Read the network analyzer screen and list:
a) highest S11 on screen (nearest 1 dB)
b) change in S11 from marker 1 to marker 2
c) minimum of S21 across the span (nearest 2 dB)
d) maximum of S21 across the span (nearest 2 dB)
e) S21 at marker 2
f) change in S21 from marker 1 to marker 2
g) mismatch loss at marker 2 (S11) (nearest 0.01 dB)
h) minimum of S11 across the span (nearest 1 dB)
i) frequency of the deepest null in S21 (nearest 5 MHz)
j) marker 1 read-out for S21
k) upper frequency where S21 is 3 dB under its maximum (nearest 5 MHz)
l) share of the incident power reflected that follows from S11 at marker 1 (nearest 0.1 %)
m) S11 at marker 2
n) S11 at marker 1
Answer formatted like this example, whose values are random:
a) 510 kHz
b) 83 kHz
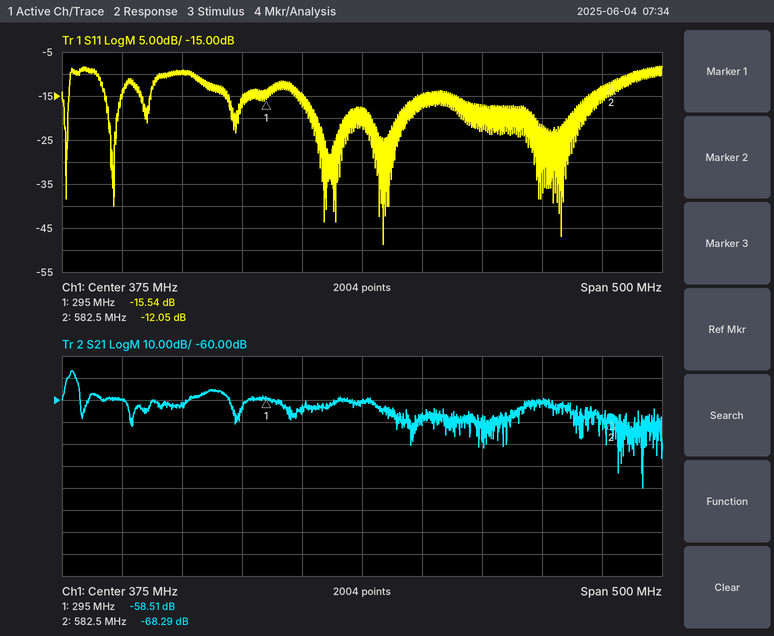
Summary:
a) -8 dB
b) 3.49 dB
c) -100 dB
d) -46 dB
e) -68.29 dB
f) -9.78 dB
g) 0.28 dB
h) -49 dB
i) 610 MHz
j) -58.51 dB
k) 135 MHz
l) 2.8 %
m) -12.05 dB
n) -15.54 dB
